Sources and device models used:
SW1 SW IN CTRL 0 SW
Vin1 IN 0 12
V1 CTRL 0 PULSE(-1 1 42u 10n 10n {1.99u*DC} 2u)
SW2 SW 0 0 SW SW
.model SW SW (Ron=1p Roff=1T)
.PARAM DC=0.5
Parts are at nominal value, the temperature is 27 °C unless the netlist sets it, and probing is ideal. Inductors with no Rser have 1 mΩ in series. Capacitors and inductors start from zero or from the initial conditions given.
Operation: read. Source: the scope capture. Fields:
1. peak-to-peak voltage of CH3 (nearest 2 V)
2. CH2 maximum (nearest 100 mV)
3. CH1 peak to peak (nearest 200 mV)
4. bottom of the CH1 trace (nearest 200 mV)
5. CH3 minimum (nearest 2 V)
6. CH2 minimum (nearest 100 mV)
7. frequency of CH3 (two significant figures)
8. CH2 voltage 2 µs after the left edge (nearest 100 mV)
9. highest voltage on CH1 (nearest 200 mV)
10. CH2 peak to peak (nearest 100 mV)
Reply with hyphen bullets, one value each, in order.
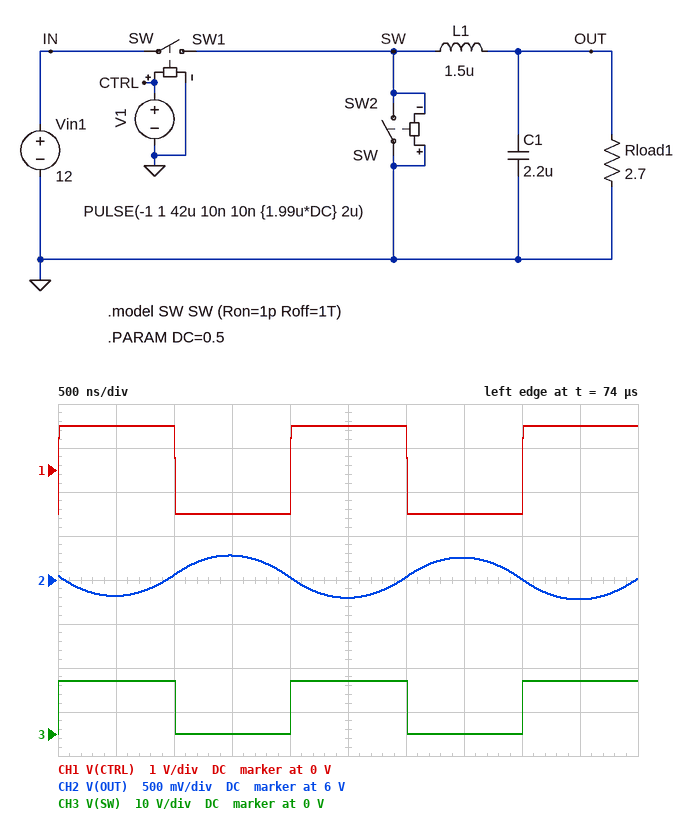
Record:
- 12 V
- 6.3 V
- 2.0 V
- -1.0 V
- 0 V
- 5.8 V
- 500 kHz
- 6.0 V
- 1.0 V
- 500 mV
